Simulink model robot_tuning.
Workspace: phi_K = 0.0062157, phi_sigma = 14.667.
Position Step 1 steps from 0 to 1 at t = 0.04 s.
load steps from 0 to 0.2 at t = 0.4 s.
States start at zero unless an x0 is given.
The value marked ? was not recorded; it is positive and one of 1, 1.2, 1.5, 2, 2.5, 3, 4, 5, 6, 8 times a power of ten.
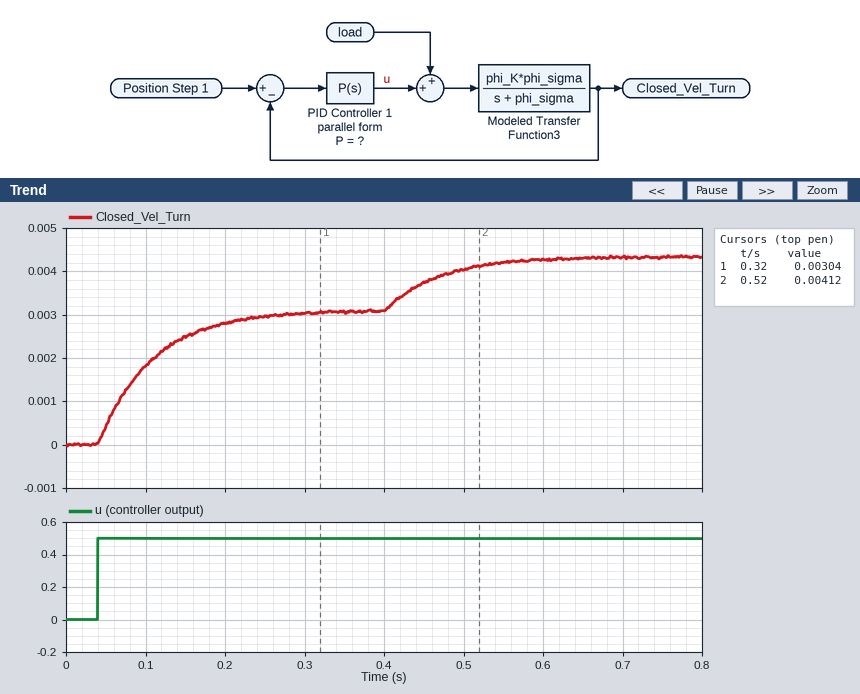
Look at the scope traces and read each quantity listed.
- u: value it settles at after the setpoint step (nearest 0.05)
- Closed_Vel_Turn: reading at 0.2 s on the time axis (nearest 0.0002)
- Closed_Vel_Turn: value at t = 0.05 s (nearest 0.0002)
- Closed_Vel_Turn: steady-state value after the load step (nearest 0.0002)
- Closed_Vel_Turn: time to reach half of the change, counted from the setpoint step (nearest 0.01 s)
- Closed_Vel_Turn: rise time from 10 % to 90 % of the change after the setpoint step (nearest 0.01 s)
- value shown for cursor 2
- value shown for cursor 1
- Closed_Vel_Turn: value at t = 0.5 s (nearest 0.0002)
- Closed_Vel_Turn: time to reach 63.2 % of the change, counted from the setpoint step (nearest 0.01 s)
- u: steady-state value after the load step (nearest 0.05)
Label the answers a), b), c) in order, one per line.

a) 0.50
b) 0.0028
c) 0.0004
d) 0.0044
e) 0.05 s
f) 0.15 s
g) 0.00412
h) 0.00304
i) 0.0040
j) 0.07 s
k) 0.50
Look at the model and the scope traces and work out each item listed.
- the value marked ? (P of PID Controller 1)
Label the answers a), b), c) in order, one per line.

a) 0.5
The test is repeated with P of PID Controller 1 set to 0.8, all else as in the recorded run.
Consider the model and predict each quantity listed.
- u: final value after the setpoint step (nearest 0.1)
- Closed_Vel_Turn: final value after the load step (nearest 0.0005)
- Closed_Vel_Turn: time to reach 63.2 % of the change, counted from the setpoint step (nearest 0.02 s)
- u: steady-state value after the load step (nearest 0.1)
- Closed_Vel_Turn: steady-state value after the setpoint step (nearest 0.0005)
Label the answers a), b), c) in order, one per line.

a) 0.8
b) 0.0060
c) 0.06 s
d) 0.8
e) 0.0050
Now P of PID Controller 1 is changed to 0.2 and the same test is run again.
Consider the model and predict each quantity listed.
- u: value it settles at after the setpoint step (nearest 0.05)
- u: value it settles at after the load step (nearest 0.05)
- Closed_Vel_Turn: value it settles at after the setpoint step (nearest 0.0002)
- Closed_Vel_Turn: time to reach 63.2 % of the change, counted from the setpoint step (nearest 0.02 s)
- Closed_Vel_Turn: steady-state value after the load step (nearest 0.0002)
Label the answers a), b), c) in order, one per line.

a) 0.20
b) 0.20
c) 0.0012
d) 0.06 s
e) 0.0024
